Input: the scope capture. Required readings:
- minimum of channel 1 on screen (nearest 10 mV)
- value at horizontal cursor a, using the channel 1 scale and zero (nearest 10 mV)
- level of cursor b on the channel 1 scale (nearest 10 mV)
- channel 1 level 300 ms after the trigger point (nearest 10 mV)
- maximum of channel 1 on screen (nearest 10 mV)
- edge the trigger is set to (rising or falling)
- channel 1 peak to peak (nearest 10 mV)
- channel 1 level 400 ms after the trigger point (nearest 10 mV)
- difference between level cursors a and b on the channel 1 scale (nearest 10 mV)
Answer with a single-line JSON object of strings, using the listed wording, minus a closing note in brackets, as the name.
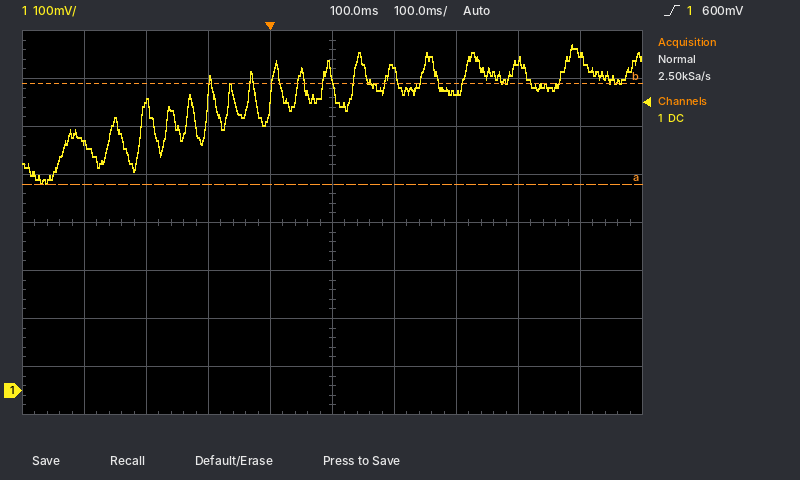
{"minimum of channel 1 on screen": "430 mV", "value at horizontal cursor a, using the channel 1 scale and zero": "430 mV", "level of cursor b on the channel 1 scale": "640 mV", "channel 1 level 300 ms after the trigger point": "620 mV", "maximum of channel 1 on screen": "720 mV", "edge the trigger is set to": "rising", "channel 1 peak to peak": "290 mV", "channel 1 level 400 ms after the trigger point": "690 mV", "difference between level cursors a and b on the channel 1 scale": "210 mV"}
